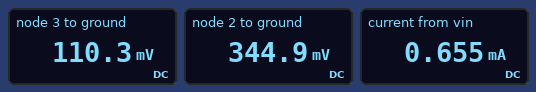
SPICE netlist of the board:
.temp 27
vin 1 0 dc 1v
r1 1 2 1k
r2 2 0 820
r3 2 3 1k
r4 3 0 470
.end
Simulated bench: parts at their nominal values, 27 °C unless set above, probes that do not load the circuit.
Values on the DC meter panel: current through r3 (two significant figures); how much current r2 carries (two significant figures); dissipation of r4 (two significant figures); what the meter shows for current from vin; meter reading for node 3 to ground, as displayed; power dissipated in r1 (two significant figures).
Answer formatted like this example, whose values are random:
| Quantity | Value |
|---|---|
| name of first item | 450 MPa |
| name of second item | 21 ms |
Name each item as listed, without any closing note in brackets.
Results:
| Quantity | Value |
|---|---|
| current through r3 | 230 µA |
| how much current r2 carries | 420 µA |
| dissipation of r4 | 26 µW |
| what the meter shows for current from vin | 0.655 mA |
| meter reading for node 3 to ground, as displayed | 110.3 mV |
| power dissipated in r1 | 430 µW |
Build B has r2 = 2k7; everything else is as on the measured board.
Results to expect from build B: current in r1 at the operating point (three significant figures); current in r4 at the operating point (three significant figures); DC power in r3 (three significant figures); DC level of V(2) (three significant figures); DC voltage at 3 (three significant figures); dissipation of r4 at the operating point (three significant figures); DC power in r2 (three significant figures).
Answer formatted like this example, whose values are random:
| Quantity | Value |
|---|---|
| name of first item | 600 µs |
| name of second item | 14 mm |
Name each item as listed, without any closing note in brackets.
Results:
| Quantity | Value |
|---|---|
| current in r1 at the operating point | 512 µA |
| current in r4 at the operating point | 332 µA |
| DC power in r3 | 110 µW |
| DC level of V(2) | 488 mV |
| DC voltage at 3 | 156 mV |
| dissipation of r4 at the operating point | 51.7 µW |
| DC power in r2 | 88.1 µW |
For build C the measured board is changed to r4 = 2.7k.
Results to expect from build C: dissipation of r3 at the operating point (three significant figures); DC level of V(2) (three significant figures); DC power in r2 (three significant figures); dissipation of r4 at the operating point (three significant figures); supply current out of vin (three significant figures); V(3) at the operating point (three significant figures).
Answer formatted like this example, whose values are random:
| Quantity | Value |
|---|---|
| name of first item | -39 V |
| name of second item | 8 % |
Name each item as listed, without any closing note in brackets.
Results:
| Quantity | Value |
|---|---|
| dissipation of r3 at the operating point | 11.8 µW |
| DC level of V(2) | 402 mV |
| DC power in r2 | 197 µW |
| dissipation of r4 at the operating point | 31.8 µW |
| supply current out of vin | 598 µA |
| V(3) at the operating point | 293 mV |
